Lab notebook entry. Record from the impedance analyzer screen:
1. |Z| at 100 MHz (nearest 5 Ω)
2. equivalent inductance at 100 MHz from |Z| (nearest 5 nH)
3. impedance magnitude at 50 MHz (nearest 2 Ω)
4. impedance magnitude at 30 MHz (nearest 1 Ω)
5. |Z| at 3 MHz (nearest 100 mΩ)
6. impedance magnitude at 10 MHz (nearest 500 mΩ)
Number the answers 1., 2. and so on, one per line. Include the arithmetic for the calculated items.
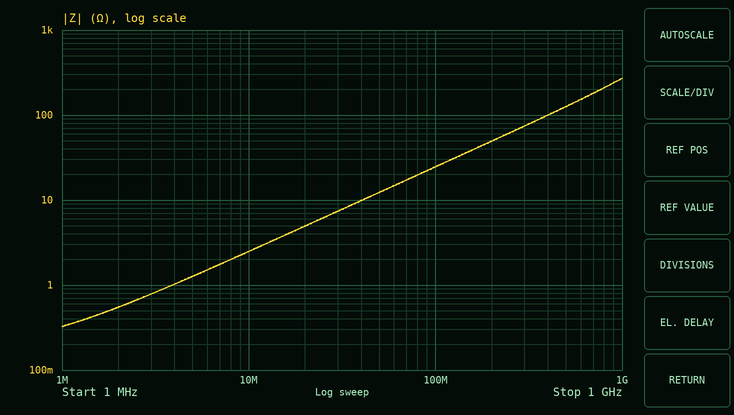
1. 25 Ω
2. L = 25 Ω/(2π × 100 MHz) ≈ 40 nH
3. 12 Ω
4. 7 Ω
5. 800 mΩ
6. 2.5 Ω
